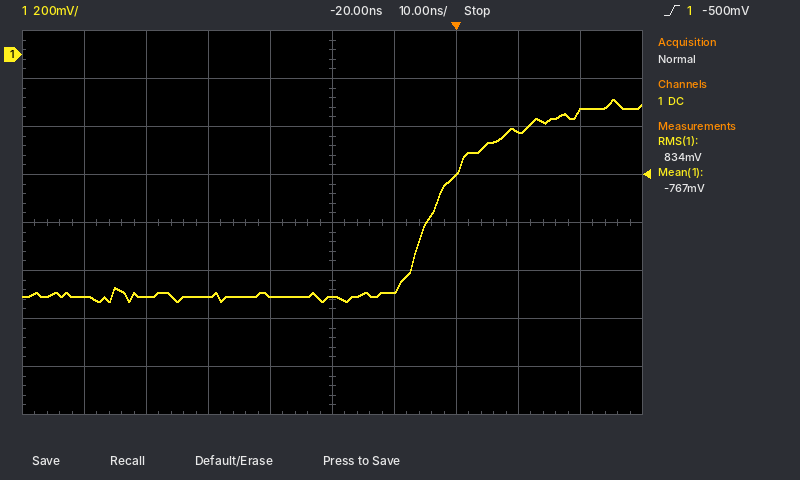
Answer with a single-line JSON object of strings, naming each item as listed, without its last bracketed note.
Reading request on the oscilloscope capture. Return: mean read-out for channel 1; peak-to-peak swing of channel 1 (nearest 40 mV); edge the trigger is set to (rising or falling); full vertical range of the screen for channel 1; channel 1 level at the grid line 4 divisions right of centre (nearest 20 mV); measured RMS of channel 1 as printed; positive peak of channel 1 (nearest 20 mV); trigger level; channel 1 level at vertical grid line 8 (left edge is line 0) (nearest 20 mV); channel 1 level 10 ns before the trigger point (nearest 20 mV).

{"mean read-out for channel 1": "-767 mV", "peak-to-peak swing of channel 1": "840 mV", "edge the trigger is set to": "rising", "full vertical range of the screen for channel 1": "1.6 V", "channel 1 level at the grid line 4 divisions right of centre": "-240 mV", "measured RMS of channel 1 as printed": "834 mV", "positive peak of channel 1": "-180 mV", "trigger level": "-500 mV", "channel 1 level at vertical grid line 8 (left edge is line 0)": "-320 mV", "channel 1 level 10 ns before the trigger point": "-980 mV"}
